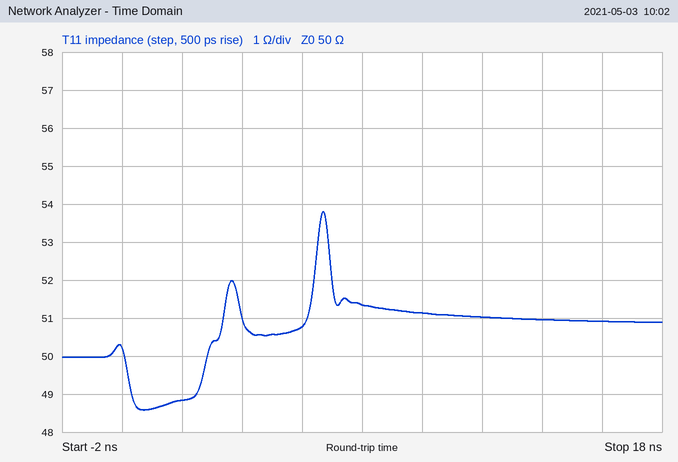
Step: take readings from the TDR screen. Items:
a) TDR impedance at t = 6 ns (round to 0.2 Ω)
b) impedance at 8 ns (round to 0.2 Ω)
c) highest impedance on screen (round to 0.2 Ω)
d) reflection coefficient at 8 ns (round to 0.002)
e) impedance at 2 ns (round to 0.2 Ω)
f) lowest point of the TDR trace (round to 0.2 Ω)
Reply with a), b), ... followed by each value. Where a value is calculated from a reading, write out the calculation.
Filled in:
a) 50.8 Ω
b) 51.4 Ω
c) 53.8 Ω
d) (51.4 − 50)/(51.4 + 50) ≈ +0.014
e) 48.8 Ω
f) 48.6 Ω
